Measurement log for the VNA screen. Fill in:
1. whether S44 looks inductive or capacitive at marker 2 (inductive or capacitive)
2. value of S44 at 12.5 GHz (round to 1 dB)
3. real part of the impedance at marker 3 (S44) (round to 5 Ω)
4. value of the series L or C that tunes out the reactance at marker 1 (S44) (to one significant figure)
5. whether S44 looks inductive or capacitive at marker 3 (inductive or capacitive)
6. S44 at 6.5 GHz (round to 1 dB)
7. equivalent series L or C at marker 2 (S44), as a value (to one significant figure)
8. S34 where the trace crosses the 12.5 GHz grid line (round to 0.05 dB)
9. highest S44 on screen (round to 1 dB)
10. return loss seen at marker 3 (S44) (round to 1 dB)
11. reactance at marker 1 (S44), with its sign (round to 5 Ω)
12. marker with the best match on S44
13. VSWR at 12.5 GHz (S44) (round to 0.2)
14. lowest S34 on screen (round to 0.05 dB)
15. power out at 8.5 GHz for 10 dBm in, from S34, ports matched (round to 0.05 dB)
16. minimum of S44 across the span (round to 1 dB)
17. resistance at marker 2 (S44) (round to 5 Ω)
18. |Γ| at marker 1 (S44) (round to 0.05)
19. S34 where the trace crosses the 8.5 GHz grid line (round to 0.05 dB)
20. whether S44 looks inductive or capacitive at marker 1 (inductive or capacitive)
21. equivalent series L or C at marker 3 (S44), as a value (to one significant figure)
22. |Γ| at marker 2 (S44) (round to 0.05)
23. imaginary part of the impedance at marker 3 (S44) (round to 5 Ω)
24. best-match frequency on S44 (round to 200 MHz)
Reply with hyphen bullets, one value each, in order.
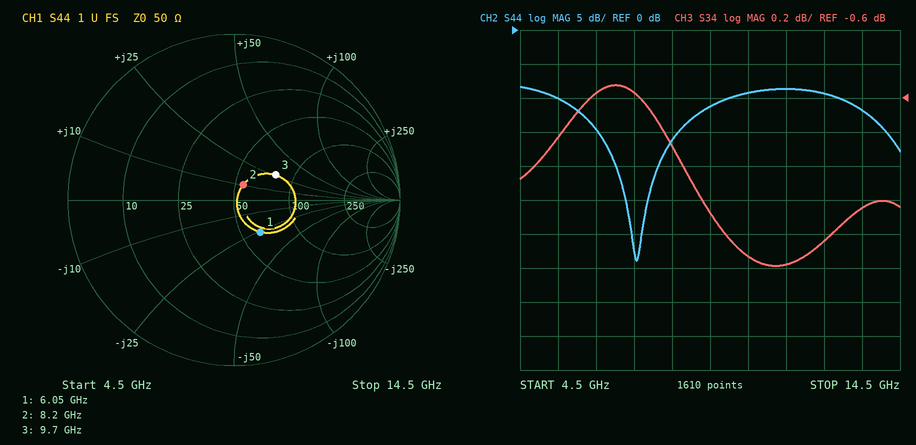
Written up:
- inductive
- -9 dB
- 80 Ω
- 700 pH
- inductive
- -15 dB
- 200 pH
- -1.45 dB
- -8 dB
- 11 dB
- -25 Ω
- marker 2
- 2.0
- -1.60 dB
- 9.10 dBm
- -34 dB
- 55 Ω
- 0.25
- -0.90 dB
- capacitive
- 400 pH
- 0.10
- +25 Ω
- 7.6 GHz
